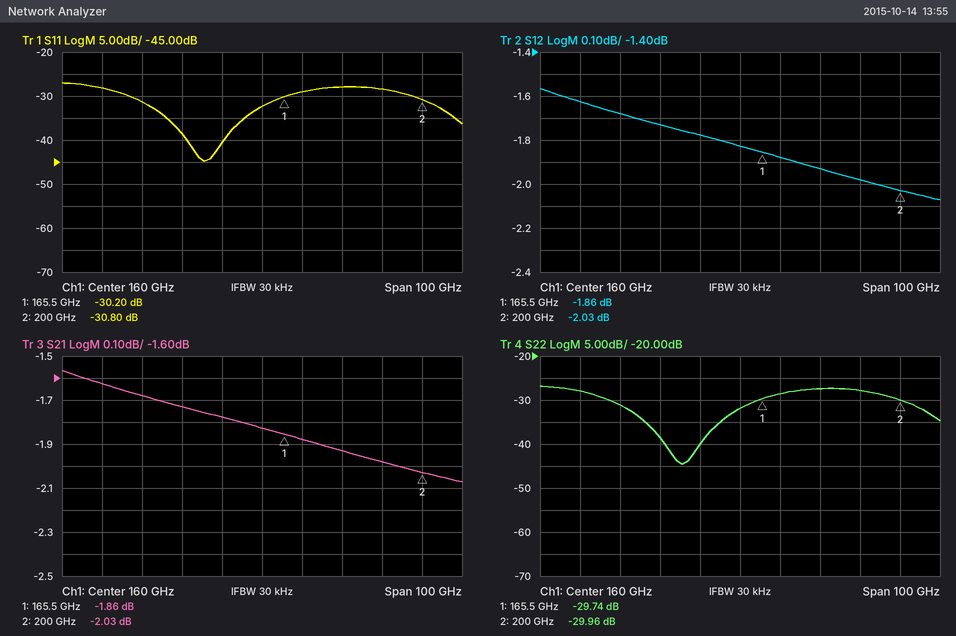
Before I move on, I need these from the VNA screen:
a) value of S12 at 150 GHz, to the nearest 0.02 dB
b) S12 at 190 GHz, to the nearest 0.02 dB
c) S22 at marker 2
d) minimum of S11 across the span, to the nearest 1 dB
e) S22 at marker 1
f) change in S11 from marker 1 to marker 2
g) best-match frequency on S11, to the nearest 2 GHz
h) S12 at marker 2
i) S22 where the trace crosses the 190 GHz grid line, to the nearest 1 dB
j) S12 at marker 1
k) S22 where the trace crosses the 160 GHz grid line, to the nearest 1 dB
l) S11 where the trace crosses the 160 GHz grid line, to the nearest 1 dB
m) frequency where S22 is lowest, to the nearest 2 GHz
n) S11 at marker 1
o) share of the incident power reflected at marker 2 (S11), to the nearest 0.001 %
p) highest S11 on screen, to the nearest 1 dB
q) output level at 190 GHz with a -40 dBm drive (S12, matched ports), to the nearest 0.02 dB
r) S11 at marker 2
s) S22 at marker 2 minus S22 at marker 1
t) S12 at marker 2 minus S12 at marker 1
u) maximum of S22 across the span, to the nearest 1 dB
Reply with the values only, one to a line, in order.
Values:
-1.78 dB
-1.98 dB
-29.96 dB
-45 dB
-29.74 dB
-0.60 dB
146 GHz
-2.03 dB
-28 dB
-1.86 dB
-32 dB
-32 dB
146 GHz
-30.20 dB
0.083 %
-27 dB
-41.98 dBm
-30.80 dB
-0.22 dB
-0.17 dB
-27 dB
